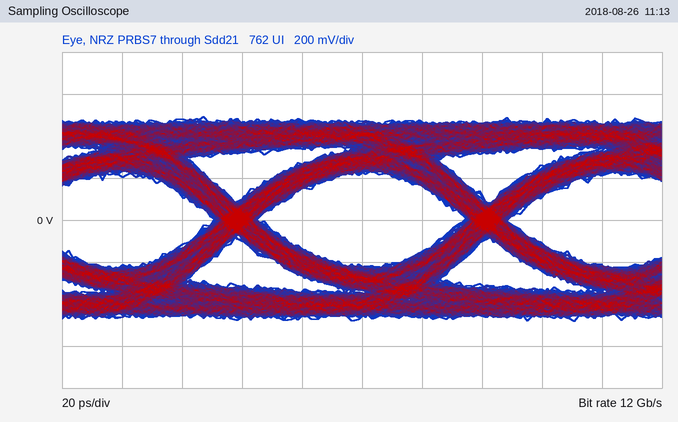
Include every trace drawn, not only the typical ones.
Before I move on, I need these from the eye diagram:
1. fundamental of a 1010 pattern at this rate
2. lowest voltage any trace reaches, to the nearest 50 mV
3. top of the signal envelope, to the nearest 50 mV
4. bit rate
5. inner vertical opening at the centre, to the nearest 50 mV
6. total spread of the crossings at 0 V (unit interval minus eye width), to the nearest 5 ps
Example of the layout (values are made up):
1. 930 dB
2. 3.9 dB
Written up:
1. 6 GHz
2. -500 mV
3. 500 mV
4. 12 Gb/s
5. 450 mV
6. 15 ps
